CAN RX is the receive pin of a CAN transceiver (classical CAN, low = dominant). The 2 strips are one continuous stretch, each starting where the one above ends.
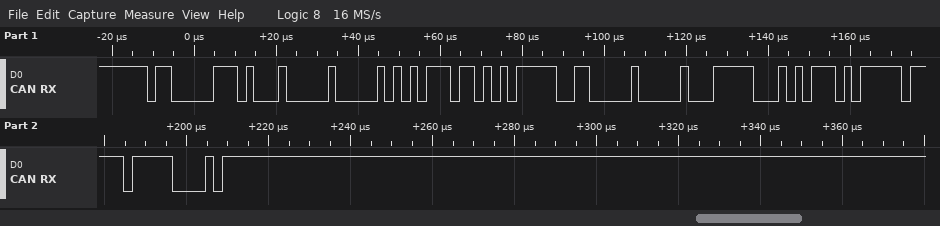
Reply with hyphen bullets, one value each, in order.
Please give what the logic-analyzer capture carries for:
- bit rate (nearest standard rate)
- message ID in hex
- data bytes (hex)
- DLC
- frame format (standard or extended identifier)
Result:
- 500 kbit/s
- 0x60D
- 00 AE D5 F6 00 0F 95 D7
- 8
- standard
